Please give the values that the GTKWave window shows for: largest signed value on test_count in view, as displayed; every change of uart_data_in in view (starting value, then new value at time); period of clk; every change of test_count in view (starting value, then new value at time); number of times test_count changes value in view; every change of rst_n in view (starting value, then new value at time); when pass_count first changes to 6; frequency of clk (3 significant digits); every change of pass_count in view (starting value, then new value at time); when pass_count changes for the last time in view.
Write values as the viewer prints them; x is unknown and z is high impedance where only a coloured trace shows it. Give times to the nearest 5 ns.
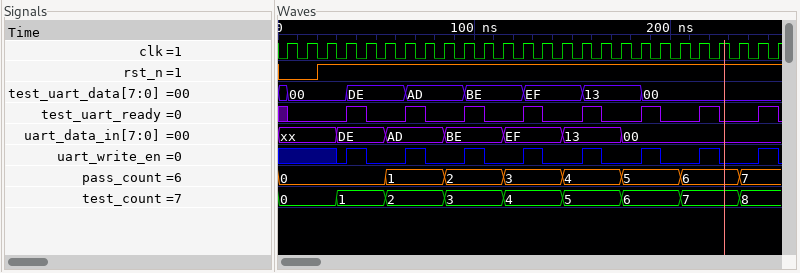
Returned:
8
xx, DE at 30 ns, AD at 55 ns, BE at 85 ns, EF at 115 ns, 13 at 145 ns, 00 at 175 ns
10 ns
0, 1 at 30 ns, 2 at 55 ns, 3 at 85 ns, 4 at 115 ns, 5 at 145 ns, 6 at 175 ns, 7 at 205 ns, 8 at 235 ns
8
0, 1 at 20 ns
205 ns
100 MHz
0, 1 at 55 ns, 2 at 85 ns, 3 at 115 ns, 4 at 145 ns, 5 at 175 ns, 6 at 205 ns, 7 at 235 ns
235 ns
